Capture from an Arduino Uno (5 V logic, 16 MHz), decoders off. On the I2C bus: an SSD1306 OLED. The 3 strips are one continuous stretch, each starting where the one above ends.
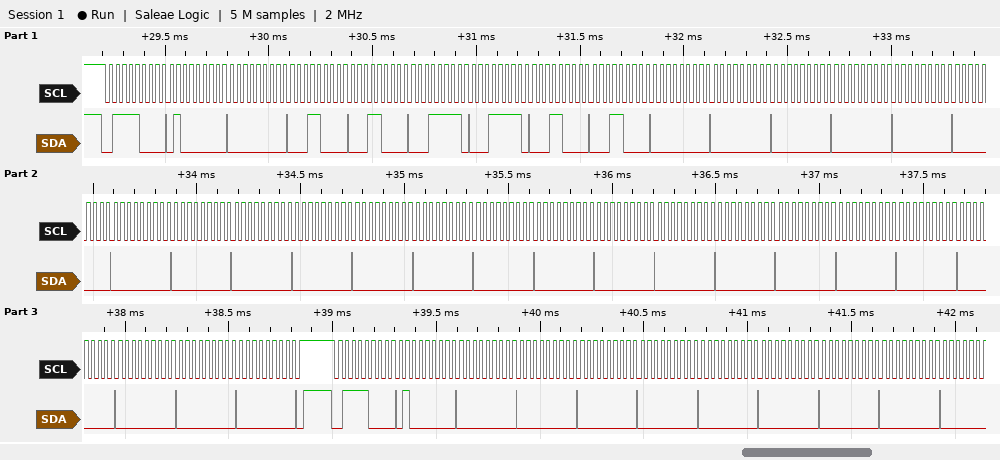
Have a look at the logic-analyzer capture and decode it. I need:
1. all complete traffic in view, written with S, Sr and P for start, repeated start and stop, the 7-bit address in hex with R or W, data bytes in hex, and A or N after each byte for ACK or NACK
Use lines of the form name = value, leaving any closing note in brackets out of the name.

all complete traffic in view, written with S, Sr and P for start, repeated start and stop, the 7-bit address in hex with R or W, data bytes in hex, and A or N after each byte for ACK or NACK = S 3CW A 40 A 00 A 18 A 18 A 1F A 1F A 18 A 18 A 00 A 00 A 00 A 00 A 00 A 00 A 00 A 00 A 00 A 00 A 00 A 00 A 00 A 00 A 00 A 00 A 00 A 00 A 00 A 00 A 00 A 00 A 00 A 00 A P S 3CW A 40 A 00 A 00 A 00 A 00 A 00 A 00 A 00 A 00 A
